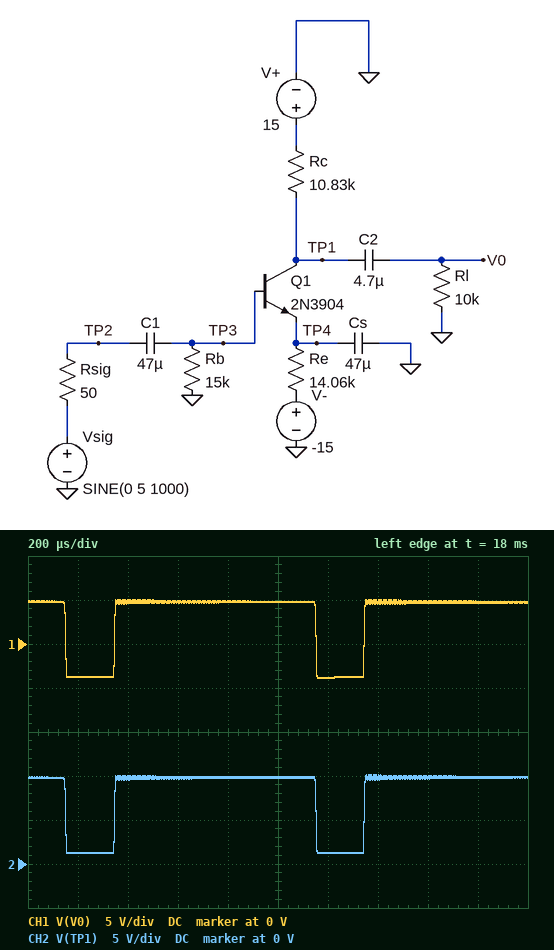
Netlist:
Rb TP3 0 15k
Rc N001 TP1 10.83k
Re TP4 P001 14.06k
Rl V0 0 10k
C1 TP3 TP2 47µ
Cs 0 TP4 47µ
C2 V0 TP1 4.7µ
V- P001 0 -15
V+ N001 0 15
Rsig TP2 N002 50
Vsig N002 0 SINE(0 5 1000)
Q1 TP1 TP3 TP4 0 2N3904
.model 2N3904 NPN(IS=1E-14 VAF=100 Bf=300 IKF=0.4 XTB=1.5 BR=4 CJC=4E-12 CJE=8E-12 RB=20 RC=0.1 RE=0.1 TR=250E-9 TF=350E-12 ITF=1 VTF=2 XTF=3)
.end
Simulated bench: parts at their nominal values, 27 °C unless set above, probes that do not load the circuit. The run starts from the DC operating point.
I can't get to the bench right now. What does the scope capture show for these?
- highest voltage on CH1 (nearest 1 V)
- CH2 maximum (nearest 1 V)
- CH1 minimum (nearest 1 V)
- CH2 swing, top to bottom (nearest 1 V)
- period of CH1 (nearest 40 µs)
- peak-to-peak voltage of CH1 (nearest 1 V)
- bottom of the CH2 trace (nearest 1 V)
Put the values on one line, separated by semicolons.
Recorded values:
5 V; 10 V; -4 V; 9 V; 1.00 ms; 9 V; 1 V
